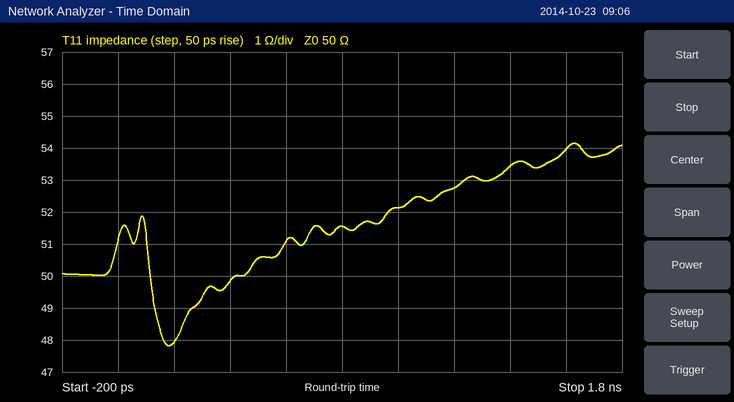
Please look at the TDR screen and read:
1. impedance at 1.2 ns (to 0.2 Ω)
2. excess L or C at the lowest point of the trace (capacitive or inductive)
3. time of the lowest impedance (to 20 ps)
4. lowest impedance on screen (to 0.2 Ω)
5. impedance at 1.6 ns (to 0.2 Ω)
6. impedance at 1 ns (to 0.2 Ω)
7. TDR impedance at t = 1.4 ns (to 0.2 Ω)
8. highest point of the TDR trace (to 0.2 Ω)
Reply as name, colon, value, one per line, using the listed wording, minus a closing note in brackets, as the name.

impedance at 1.2 ns: 52.8 Ω
excess L or C at the lowest point of the trace: capacitive
time of the lowest impedance: 180 ps
lowest impedance on screen: 47.8 Ω
impedance at 1.6 ns: 54.0 Ω
impedance at 1 ns: 52.2 Ω
TDR impedance at t = 1.4 ns: 53.4 Ω
highest point of the TDR trace: 54.2 Ω
